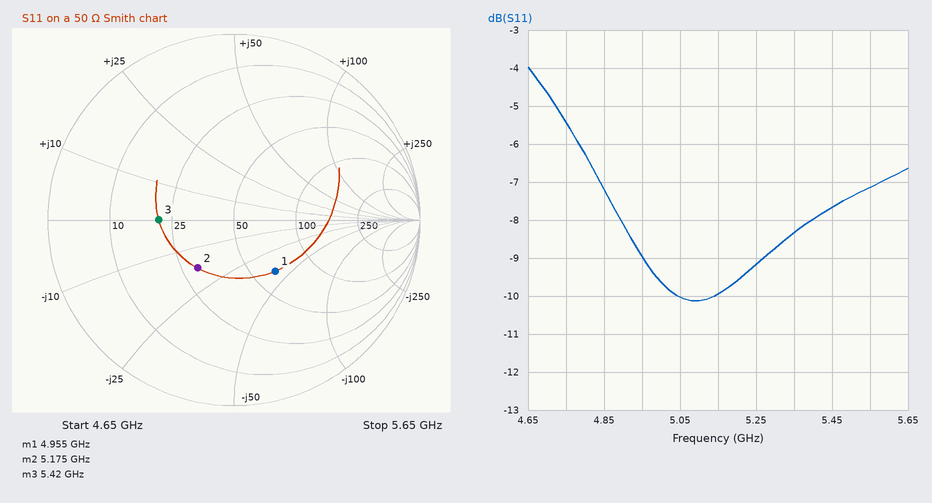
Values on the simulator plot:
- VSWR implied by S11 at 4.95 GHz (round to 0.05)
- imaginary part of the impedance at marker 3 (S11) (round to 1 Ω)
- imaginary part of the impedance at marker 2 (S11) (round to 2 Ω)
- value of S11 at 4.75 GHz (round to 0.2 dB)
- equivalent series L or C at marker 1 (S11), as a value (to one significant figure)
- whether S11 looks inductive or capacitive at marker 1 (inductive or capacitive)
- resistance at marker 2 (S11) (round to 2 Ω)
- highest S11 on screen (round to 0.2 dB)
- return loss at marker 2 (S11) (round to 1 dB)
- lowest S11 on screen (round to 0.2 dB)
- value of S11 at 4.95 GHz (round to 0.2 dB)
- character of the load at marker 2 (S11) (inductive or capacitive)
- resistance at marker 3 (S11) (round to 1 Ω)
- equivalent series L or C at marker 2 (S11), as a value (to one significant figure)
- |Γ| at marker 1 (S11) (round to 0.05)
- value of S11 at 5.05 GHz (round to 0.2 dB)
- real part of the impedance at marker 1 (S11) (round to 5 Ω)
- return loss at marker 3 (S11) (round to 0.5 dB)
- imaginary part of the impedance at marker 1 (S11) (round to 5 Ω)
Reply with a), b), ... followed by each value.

a) 2.10
b) 0 Ω
c) -18 Ω
d) -5.4 dB
e) 800 fF
f) capacitive
g) 30 Ω
h) -4.0 dB
i) 10 dB
j) -10.2 dB
k) -9.0 dB
l) capacitive
m) 21 Ω
n) 2 pF
o) 0.35
p) -10.0 dB
q) 65 Ω
r) 8.0 dB
s) -40 Ω
